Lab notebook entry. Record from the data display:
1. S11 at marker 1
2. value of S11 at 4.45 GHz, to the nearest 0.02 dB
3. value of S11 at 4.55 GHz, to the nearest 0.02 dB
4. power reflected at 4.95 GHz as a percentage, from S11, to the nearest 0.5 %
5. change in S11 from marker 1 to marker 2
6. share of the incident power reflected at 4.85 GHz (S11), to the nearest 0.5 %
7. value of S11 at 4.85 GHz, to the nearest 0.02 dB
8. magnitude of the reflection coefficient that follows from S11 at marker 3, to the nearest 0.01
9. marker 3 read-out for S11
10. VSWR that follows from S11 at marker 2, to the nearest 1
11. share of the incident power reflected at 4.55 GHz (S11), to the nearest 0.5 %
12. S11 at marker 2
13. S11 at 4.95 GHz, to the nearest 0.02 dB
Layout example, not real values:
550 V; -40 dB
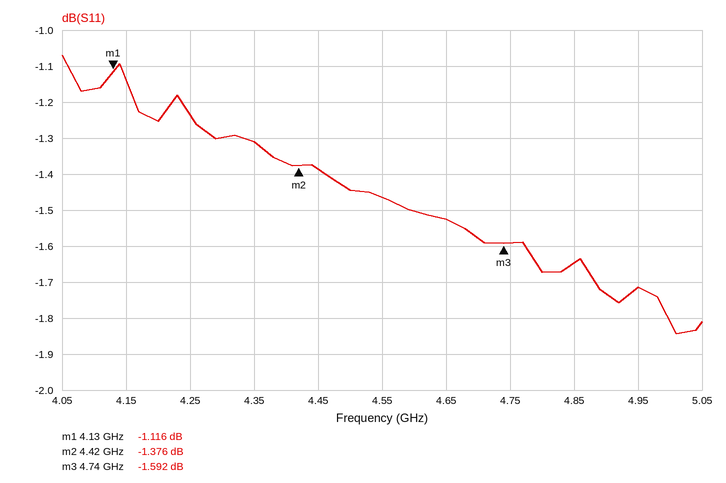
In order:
-1.116 dB; -1.38 dB; -1.46 dB; 67.5 %; -0.260 dB; 68.5 %; -1.64 dB; 0.83; -1.592 dB; 13; 71.5 %; -1.376 dB; -1.72 dB
